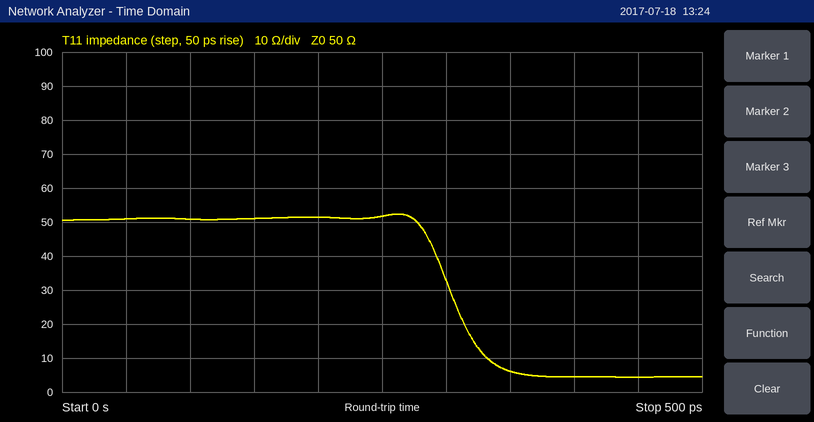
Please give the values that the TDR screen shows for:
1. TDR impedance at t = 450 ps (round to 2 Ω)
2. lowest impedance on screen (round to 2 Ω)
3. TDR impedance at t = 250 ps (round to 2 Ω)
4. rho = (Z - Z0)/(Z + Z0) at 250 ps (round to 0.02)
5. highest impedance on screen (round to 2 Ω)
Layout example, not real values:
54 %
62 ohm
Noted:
4 Ω
4 Ω
52 Ω
+0.02
52 Ω
